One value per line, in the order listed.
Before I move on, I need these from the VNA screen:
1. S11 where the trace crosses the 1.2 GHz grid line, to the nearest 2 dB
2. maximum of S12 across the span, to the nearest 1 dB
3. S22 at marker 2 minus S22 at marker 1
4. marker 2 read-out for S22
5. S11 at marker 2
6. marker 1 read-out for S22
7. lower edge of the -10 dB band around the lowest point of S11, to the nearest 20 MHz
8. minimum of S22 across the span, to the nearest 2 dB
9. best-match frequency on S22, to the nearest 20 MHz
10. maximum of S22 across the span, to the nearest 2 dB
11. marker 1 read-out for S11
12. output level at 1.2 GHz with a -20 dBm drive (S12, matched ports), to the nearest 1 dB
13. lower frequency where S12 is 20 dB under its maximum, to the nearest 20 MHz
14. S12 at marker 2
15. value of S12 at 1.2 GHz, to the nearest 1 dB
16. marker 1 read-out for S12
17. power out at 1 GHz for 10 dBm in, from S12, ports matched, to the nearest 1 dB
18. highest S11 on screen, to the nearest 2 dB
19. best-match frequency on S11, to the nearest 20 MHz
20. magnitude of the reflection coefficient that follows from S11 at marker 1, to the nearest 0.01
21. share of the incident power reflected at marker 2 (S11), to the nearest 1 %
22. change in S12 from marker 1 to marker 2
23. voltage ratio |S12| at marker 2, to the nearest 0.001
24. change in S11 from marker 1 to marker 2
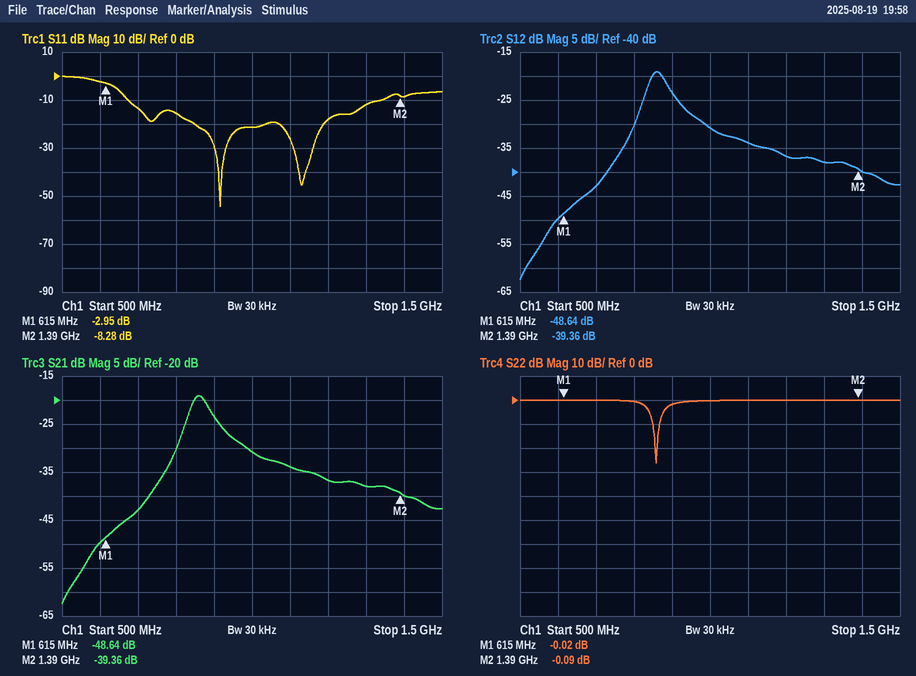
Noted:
-18 dB
-19 dB
-0.07 dB
-0.09 dB
-8.28 dB
-0.02 dB
680 MHz
-26 dB
860 MHz
0 dB
-2.95 dB
-57 dBm
740 MHz
-39.36 dB
-37 dB
-48.64 dB
-21 dBm
0 dB
920 MHz
0.71
15 %
9.28 dB
0.011
-5.33 dB
